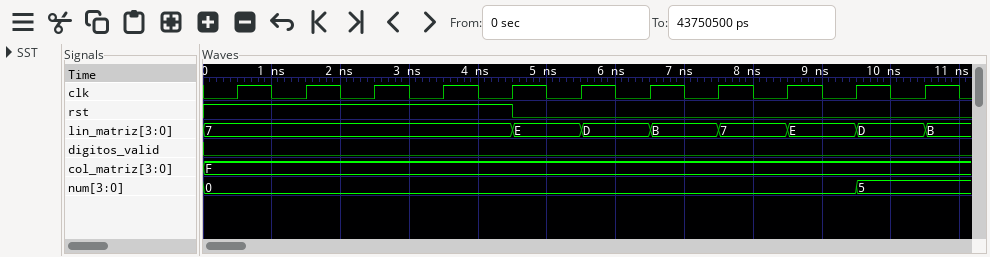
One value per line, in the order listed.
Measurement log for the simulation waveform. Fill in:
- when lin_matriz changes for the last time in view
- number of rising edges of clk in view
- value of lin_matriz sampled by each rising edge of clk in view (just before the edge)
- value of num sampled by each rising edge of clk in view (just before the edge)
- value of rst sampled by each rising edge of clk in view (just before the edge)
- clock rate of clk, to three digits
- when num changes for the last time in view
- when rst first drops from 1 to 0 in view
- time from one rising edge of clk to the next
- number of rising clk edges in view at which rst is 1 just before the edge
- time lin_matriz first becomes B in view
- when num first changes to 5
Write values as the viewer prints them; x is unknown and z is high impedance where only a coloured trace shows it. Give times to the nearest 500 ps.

10500 ps
11
7, 7, 7, 7, 7, E, D, B, 7, E, D
0, 0, 0, 0, 0, 0, 0, 0, 0, 0, 5
1 1 1 1 1 0 0 0 0 0 0
1.00 GHz
9500 ps
4500 ps
1000 ps
5
6500 ps
9500 ps
